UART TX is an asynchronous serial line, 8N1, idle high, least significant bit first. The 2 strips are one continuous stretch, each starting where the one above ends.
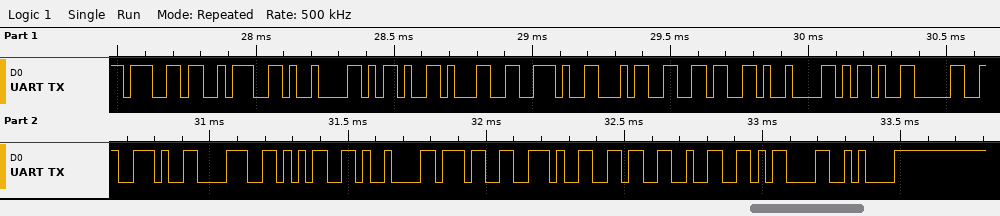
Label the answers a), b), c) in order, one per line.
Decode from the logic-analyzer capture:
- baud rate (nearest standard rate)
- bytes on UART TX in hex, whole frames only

a) 38400 baud
b) 0x67 0x3A 0x09 0x2D 0x31 0x2E 0x34 0x36 0x09 0x2D 0x30 0x2E 0x38 0x35 0x09 0x37 0x2E 0x36 0x32 0x0D 0x0A
